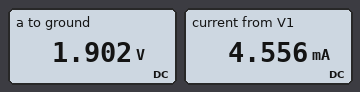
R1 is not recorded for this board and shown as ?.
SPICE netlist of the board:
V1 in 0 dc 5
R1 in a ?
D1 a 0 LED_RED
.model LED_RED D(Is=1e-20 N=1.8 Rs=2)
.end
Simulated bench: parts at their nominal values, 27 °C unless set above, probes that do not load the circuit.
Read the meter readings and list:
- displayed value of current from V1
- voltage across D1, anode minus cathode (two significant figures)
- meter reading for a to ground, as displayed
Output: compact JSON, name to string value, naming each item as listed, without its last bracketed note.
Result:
{"displayed value of current from V1": "4.556 mA", "voltage across D1, anode minus cathode": "1.9 V", "meter reading for a to ground, as displayed": "1.902 V"}
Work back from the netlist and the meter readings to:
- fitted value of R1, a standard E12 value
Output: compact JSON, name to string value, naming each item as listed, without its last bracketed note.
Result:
{"fitted value of R1, a standard E12 value": "680 Ω"}
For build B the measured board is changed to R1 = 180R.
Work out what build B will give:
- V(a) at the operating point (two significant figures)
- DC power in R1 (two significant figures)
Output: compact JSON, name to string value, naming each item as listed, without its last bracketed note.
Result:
{"V(a) at the operating point": "2.0 V", "DC power in R1": "50 mW"}
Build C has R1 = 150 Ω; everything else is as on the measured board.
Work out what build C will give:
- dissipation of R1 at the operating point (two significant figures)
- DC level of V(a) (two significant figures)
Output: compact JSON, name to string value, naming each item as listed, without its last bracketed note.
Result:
{"dissipation of R1 at the operating point": "60 mW", "DC level of V(a)": "2.0 V"}
